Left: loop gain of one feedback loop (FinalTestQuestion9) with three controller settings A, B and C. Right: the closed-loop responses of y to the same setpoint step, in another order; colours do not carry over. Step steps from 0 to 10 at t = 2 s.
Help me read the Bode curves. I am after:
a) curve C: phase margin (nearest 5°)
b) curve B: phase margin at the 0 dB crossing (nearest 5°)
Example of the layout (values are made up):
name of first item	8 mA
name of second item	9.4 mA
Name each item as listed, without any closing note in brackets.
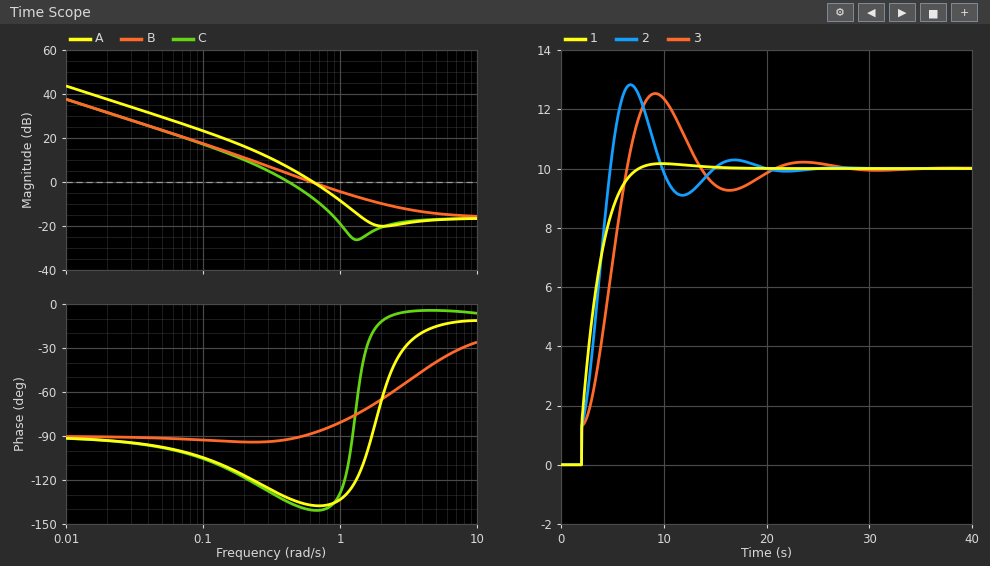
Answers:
curve C: phase margin	45°
curve B: phase margin at the 0 dB crossing	90°
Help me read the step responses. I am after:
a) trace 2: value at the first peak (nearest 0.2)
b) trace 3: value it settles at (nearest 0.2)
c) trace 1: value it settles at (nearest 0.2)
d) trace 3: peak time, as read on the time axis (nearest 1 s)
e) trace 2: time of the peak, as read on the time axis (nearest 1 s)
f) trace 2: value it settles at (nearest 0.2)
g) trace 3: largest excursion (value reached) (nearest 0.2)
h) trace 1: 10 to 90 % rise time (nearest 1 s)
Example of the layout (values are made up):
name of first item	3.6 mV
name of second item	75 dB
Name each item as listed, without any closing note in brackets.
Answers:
trace 2: value at the first peak	12.8
trace 3: value it settles at	10.0
trace 1: value it settles at	10.0
trace 3: peak time, as read on the time axis	9 s
trace 2: time of the peak, as read on the time axis	7 s
trace 2: value it settles at	10.0
trace 3: largest excursion (value reached)	12.6
trace 1: 10 to 90 % rise time	3 s
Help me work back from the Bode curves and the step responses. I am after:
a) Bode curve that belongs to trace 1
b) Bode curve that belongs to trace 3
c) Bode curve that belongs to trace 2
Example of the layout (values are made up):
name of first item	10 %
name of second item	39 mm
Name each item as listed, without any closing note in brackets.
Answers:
Bode curve that belongs to trace 1	B
Bode curve that belongs to trace 3	C
Bode curve that belongs to trace 2	A
